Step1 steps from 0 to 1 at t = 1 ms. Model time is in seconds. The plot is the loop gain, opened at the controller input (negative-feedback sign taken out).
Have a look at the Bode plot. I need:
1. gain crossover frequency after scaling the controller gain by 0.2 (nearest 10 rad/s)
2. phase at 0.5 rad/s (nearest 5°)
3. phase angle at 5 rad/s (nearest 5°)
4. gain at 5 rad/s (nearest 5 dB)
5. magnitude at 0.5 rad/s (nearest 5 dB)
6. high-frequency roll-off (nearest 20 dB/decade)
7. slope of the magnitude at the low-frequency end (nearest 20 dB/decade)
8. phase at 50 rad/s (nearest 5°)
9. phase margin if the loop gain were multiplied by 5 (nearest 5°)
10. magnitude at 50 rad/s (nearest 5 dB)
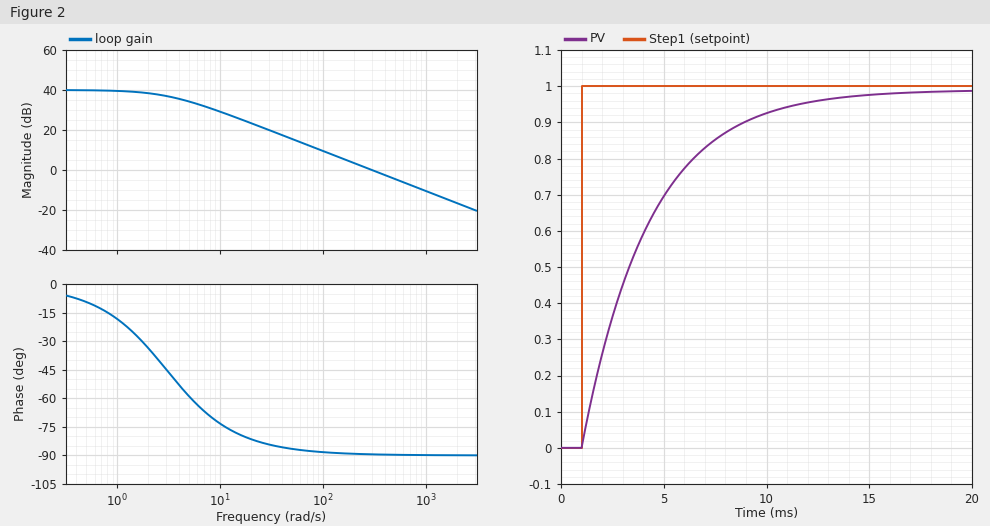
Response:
60 rad/s
-10°
-60°
35 dB
40 dB
-20 dB/decade
0 dB/decade
-85°
90°
15 dB
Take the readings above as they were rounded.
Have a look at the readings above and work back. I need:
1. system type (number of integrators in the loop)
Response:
0
